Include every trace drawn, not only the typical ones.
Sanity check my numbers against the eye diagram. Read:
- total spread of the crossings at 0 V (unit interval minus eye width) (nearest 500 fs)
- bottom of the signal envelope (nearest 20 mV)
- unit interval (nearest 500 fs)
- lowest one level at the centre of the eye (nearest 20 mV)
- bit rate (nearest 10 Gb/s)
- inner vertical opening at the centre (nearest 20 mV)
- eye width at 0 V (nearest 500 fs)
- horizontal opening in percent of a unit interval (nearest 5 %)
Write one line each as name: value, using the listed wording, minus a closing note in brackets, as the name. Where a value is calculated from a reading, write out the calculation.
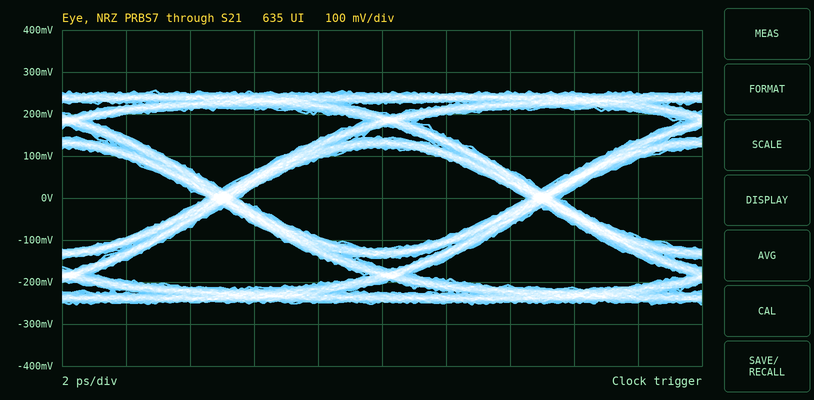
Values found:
total spread of the crossings at 0 V (unit interval minus eye width): 1.0 ps
bottom of the signal envelope: -260 mV
unit interval: 10.0 ps
lowest one level at the centre of the eye: 120 mV
bit rate: 100 Gb/s
inner vertical opening at the centre: 240 mV
eye width at 0 V: 9.0 ps
horizontal opening in percent of a unit interval: 9.0 ps / 10.0 ps ≈ 90 %
